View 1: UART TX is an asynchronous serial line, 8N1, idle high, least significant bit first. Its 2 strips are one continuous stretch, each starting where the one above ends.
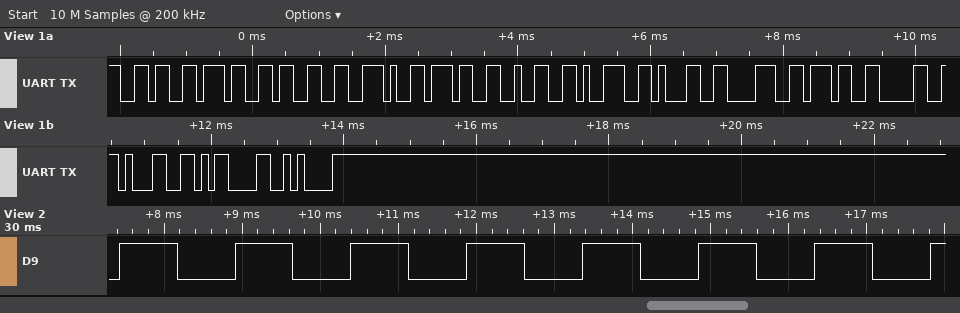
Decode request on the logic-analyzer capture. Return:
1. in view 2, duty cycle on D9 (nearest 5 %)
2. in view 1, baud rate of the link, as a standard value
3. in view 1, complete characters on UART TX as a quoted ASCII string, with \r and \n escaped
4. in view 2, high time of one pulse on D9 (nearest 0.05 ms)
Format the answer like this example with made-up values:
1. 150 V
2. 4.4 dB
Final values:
1. 50 %
2. 9600 baud
3. "673.72918701\r\n"
4. 0.75 ms
